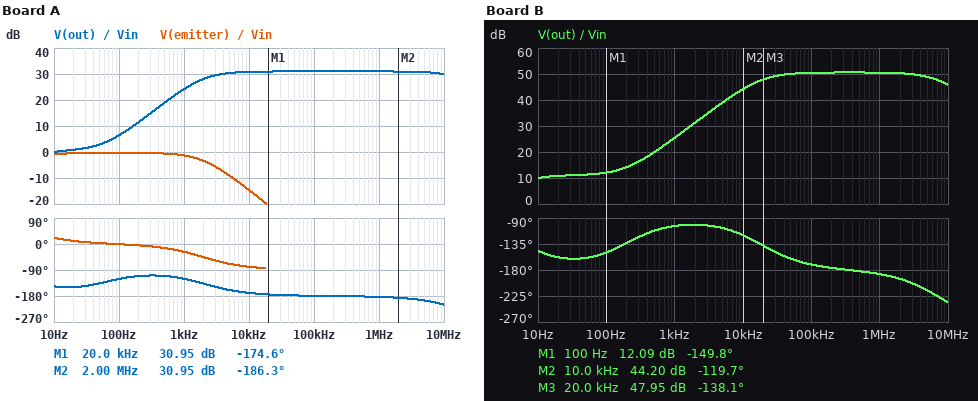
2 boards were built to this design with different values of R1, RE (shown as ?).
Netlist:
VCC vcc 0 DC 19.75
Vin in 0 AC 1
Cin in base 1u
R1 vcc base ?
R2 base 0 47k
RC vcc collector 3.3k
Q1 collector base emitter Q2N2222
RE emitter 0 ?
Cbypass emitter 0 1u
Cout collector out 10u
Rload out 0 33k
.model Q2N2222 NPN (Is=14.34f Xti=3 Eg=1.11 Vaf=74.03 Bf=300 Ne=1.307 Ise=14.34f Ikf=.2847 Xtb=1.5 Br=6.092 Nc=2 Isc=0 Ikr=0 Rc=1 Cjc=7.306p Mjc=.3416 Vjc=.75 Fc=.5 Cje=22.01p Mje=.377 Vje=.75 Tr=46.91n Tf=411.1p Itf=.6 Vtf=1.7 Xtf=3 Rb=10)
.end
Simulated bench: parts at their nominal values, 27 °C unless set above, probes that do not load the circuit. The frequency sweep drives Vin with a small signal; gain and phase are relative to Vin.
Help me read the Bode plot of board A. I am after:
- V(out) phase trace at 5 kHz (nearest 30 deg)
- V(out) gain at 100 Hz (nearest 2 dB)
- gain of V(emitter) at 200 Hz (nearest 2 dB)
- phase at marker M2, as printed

-150 deg
6 dB
0 dB
-186.3 deg
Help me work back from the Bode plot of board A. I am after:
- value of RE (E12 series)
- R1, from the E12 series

2.7 kΩ
560 kΩ
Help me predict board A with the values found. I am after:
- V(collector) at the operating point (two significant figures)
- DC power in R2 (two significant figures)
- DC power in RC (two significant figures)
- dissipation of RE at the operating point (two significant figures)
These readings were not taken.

19 V
45 µW
320 µW
260 µW
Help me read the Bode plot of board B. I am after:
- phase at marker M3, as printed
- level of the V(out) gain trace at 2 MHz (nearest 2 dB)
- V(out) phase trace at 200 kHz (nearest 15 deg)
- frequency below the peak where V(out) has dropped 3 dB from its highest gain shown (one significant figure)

-138.1 deg
50 dB
-180 deg
20 kHz
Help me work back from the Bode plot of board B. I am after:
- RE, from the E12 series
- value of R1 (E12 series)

820 Ω
180 kΩ
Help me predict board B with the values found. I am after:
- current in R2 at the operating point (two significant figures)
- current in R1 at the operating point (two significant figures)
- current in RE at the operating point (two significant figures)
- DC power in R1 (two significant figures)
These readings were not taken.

73 µA
91 µA
3.4 mA
1.5 mW
